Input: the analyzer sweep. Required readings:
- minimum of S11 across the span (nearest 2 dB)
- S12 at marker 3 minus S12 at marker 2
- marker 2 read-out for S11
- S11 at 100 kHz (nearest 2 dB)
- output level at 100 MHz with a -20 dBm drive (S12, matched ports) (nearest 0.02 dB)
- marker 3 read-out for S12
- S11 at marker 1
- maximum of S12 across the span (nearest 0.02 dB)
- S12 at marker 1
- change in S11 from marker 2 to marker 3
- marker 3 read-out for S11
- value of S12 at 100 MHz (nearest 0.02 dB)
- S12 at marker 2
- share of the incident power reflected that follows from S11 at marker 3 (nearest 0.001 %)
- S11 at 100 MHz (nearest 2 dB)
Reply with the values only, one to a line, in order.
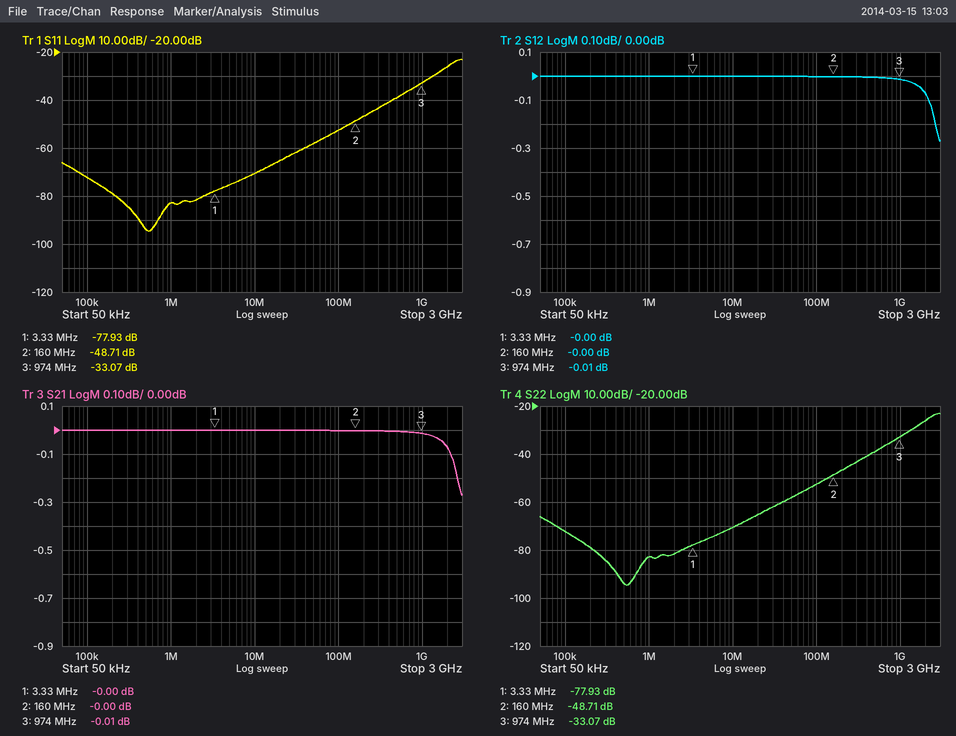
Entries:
-94 dB
-0.01 dB
-48.71 dB
-72 dB
-20.00 dBm
-0.01 dB
-77.93 dB
0.00 dB
-0.00 dB
15.64 dB
-33.07 dB
0.00 dB
-0.00 dB
0.049 %
-52 dB
